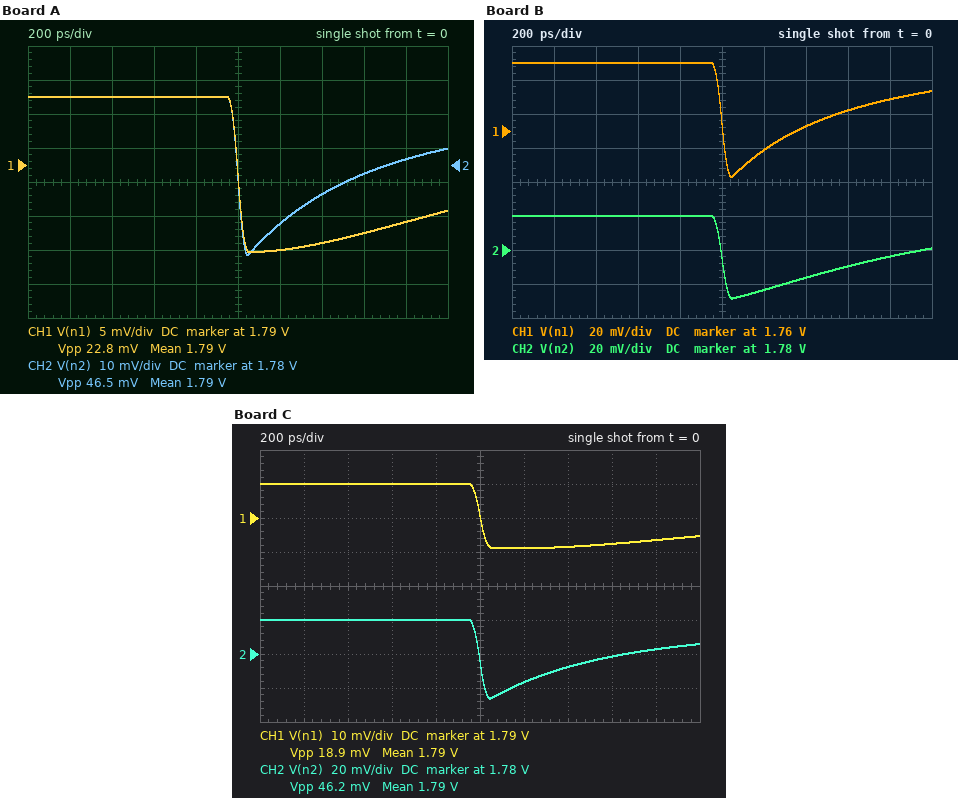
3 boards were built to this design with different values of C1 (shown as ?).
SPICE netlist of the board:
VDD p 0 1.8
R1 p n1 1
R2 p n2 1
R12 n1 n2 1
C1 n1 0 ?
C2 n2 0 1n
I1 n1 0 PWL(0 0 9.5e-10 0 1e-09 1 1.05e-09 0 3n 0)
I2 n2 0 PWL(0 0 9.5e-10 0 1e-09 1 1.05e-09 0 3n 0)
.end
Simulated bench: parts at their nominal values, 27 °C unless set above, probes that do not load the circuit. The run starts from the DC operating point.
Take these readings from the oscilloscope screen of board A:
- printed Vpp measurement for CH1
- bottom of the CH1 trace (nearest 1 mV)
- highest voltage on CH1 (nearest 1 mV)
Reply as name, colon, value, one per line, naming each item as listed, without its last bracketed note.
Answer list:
printed Vpp measurement for CH1: 22.8 mV
bottom of the CH1 trace: 1.777 V
highest voltage on CH1: 1.800 V
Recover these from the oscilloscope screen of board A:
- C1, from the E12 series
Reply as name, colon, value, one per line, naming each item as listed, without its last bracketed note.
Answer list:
C1, from the E12 series: 2.2 nF
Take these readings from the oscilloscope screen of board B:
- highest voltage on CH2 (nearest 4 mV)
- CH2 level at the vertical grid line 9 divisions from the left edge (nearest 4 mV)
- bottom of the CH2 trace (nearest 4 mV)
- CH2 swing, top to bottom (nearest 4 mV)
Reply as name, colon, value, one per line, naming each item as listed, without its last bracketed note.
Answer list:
highest voltage on CH2: 1.800 V
CH2 level at the vertical grid line 9 divisions from the left edge: 1.776 V
bottom of the CH2 trace: 1.752 V
CH2 swing, top to bottom: 48 mV
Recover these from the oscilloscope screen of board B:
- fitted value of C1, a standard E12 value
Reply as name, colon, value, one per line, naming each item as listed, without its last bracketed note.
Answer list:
fitted value of C1, a standard E12 value: 680 pF
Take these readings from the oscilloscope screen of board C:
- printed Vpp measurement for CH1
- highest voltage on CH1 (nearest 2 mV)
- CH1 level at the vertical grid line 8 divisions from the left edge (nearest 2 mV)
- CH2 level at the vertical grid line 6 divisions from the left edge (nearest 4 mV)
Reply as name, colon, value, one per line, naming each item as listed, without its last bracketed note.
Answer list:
printed Vpp measurement for CH1: 18.9 mV
highest voltage on CH1: 1.800 V
CH1 level at the vertical grid line 8 divisions from the left edge: 1.782 V
CH2 level at the vertical grid line 6 divisions from the left edge: 1.764 V
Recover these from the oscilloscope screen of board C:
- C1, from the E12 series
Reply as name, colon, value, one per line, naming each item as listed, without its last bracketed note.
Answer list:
C1, from the E12 series: 2.7 nF
